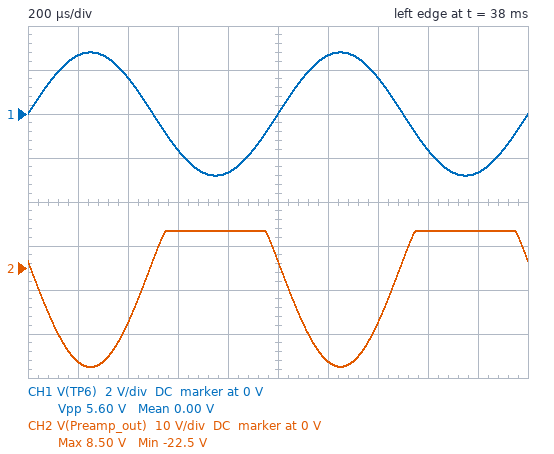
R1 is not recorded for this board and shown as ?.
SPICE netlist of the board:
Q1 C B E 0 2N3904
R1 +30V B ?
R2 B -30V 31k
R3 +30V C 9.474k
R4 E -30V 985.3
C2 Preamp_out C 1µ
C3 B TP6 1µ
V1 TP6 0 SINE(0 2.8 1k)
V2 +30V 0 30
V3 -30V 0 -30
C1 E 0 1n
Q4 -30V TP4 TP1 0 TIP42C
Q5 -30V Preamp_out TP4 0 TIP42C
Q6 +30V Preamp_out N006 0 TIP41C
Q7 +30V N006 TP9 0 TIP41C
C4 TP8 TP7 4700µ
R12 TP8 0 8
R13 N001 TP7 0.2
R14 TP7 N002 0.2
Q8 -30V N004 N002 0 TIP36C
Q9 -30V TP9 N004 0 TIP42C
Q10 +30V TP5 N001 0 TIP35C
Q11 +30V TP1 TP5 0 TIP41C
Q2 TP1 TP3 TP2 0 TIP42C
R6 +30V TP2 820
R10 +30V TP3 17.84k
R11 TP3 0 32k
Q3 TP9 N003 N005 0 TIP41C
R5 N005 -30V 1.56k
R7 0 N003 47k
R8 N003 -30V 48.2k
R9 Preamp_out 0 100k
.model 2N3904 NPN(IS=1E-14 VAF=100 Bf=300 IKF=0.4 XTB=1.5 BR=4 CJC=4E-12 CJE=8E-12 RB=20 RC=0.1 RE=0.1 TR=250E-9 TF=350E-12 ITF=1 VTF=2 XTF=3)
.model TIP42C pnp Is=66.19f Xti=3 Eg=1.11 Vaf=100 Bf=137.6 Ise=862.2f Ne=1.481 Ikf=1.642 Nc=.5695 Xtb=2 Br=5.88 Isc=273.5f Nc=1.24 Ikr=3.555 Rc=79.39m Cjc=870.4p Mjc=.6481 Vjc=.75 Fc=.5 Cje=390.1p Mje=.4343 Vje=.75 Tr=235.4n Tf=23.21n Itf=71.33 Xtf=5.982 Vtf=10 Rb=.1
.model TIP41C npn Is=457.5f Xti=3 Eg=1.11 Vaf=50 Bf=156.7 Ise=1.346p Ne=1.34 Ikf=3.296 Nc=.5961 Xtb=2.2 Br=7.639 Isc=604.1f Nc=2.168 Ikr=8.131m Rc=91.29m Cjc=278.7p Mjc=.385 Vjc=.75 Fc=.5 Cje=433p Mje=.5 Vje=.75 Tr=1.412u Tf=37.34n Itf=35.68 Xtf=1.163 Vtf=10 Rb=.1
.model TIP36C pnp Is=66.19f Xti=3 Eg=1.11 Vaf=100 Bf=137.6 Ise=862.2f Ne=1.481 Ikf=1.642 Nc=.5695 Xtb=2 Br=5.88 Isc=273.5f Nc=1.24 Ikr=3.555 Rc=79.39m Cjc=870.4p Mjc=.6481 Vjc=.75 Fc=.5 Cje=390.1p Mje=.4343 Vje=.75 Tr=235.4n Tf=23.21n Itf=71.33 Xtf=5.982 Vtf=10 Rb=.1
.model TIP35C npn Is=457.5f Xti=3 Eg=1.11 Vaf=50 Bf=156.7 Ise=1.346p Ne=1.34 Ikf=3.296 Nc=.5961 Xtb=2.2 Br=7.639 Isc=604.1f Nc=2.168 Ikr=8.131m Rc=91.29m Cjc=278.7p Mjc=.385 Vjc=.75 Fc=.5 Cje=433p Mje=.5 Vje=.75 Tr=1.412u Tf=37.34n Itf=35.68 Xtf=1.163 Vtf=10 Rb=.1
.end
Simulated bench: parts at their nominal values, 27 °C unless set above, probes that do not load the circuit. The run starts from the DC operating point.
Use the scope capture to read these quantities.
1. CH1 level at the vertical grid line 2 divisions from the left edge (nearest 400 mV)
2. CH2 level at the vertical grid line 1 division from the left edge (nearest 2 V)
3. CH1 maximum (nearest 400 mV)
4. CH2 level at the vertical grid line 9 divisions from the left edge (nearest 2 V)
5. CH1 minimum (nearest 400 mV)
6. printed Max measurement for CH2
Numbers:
1.6 V
-22 V
2.8 V
8 V
-2.8 V
8.50 V
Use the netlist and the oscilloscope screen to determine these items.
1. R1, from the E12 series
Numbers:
1.2 MΩ
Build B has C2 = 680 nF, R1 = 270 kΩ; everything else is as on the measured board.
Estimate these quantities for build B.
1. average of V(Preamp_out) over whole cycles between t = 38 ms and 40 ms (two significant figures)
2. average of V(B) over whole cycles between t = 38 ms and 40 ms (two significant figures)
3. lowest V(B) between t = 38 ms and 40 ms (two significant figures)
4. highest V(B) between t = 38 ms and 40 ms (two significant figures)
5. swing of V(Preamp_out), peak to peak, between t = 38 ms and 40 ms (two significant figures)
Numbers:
7.4 V
-26 V
-29 V
-23 V
44 V
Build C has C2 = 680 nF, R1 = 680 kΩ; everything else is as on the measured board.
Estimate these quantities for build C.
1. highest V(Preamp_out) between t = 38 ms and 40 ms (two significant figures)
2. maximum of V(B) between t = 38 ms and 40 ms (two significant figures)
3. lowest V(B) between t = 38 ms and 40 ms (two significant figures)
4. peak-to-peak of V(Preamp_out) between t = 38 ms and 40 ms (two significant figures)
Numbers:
17 V
-25 V
-30 V
40 V
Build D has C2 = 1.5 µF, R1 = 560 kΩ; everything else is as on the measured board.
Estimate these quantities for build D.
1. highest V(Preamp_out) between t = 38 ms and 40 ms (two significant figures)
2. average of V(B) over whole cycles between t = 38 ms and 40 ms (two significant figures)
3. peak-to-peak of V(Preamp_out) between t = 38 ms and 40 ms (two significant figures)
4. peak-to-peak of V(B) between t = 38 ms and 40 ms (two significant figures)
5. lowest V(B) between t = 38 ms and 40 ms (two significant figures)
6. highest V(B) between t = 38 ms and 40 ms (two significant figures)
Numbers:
20 V
-27 V
44 V
5.6 V
-30 V
-24 V
